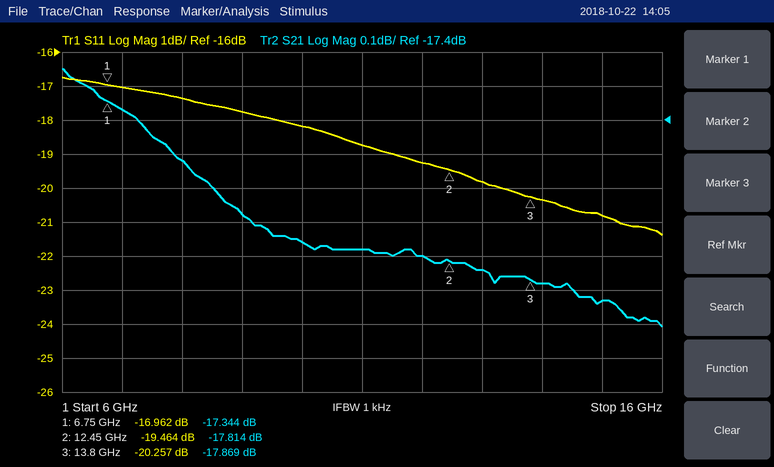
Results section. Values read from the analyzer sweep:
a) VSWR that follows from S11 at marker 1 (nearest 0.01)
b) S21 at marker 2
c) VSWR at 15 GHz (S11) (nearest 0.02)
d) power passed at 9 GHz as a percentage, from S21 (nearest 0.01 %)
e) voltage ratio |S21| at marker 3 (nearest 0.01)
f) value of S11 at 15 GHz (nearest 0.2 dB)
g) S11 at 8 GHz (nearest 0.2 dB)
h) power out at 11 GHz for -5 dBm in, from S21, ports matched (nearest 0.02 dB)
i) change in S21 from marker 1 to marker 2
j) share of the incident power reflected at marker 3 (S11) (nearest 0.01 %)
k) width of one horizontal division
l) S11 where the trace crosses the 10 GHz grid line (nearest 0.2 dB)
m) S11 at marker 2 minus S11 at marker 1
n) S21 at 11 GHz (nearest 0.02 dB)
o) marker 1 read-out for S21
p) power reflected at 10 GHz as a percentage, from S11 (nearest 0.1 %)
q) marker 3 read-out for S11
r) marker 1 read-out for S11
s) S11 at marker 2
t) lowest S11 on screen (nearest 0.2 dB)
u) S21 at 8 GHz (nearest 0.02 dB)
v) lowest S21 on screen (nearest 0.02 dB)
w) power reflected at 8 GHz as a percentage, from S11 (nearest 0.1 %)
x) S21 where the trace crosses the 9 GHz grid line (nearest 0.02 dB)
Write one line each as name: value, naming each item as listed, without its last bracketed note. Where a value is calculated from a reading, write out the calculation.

VSWR that follows from S11 at marker 1: (1 + 0.1419)/(1 − 0.1419) ≈ 1.33
S21 at marker 2: -17.814 dB
VSWR at 15 GHz (S11): |Γ| = 10^(-20.8/20) = 0.0912; VSWR = (1 + 0.0912)/(1 − 0.0912) ≈ 1.20
power passed at 9 GHz as a percentage, from S21: 10^(-17.68/10) ≈ 1.71 %
voltage ratio |S21| at marker 3: 10^(-17.869/20) ≈ 0.13
value of S11 at 15 GHz: -20.8 dB
S11 at 8 GHz: -17.4 dB
power out at 11 GHz for -5 dBm in, from S21, ports matched: -5 dBm + (-17.78 dB) = -22.78 dBm
change in S21 from marker 1 to marker 2: -17.814 − (-17.344) = -0.470 dB
share of the incident power reflected at marker 3 (S11): 10^(-20.257/10) ≈ 0.94 %
width of one horizontal division: 1 GHz
S11 where the trace crosses the 10 GHz grid line: -18.2 dB
S11 at marker 2 minus S11 at marker 1: -19.464 − (-16.962) = -2.502 dB
S21 at 11 GHz: -17.78 dB
marker 1 read-out for S21: -17.344 dB
power reflected at 10 GHz as a percentage, from S11: 10^(-18.2/10) ≈ 1.5 %
marker 3 read-out for S11: -20.257 dB
marker 1 read-out for S11: -16.962 dB
S11 at marker 2: -19.464 dB
lowest S11 on screen: -21.4 dB
S21 at 8 GHz: -17.52 dB
lowest S21 on screen: -18.00 dB
power reflected at 8 GHz as a percentage, from S11: 10^(-17.4/10) ≈ 1.8 %
S21 where the trace crosses the 9 GHz grid line: -17.68 dB
